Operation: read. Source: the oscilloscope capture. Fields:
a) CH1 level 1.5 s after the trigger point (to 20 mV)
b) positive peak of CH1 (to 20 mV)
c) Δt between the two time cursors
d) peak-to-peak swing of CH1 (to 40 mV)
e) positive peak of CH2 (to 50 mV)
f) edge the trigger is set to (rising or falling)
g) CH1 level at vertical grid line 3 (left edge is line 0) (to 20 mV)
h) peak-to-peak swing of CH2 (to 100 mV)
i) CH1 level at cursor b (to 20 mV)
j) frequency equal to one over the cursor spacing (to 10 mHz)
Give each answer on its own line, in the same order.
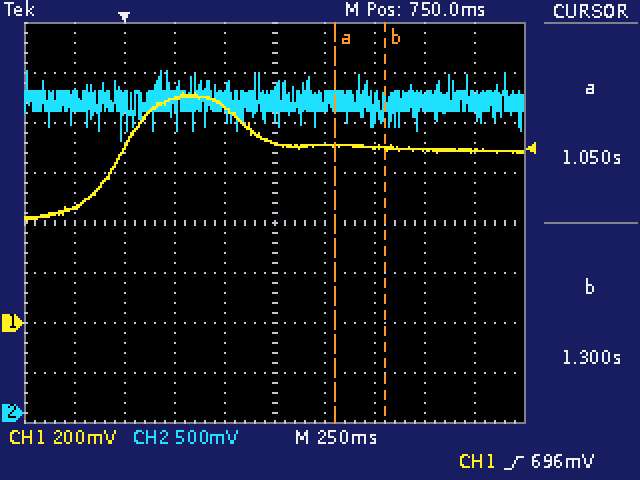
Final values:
700 mV
920 mV
250 ms
520 mV
3.40 V
rising
900 mV
700 mV
700 mV
4.00 Hz
